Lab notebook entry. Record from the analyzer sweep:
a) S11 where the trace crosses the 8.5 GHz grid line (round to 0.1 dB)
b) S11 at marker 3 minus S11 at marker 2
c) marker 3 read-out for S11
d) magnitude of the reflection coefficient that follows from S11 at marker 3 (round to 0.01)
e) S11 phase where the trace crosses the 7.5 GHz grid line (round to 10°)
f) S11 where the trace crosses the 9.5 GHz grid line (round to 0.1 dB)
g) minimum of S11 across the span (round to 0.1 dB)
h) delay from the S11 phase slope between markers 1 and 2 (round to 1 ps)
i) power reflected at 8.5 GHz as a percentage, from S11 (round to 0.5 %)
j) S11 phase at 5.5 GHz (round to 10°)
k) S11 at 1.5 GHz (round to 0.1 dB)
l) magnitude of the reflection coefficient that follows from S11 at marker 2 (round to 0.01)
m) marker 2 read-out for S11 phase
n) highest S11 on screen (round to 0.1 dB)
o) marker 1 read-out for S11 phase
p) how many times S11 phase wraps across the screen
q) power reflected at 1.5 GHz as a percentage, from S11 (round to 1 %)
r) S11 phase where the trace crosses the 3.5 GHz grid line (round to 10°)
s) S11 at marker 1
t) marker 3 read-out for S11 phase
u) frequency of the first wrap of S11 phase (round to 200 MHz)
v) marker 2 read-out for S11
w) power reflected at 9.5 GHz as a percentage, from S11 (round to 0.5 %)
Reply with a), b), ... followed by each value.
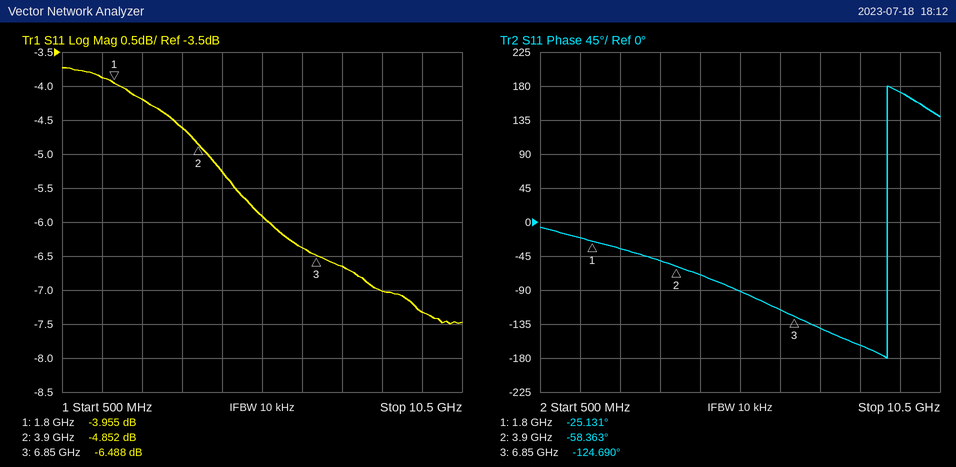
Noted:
a) -7.0 dB
b) -1.636 dB
c) -6.488 dB
d) 0.47
e) -140°
f) -7.3 dB
g) -7.5 dB
h) 44 ps
i) 20.0 %
j) -90°
k) -3.9 dB
l) 0.57
m) -58.363°
n) -3.7 dB
o) -25.131°
p) 1
q) 41 %
r) -50°
s) -3.955 dB
t) -124.690°
u) 9.2 GHz
v) -4.852 dB
w) 18.5 %
